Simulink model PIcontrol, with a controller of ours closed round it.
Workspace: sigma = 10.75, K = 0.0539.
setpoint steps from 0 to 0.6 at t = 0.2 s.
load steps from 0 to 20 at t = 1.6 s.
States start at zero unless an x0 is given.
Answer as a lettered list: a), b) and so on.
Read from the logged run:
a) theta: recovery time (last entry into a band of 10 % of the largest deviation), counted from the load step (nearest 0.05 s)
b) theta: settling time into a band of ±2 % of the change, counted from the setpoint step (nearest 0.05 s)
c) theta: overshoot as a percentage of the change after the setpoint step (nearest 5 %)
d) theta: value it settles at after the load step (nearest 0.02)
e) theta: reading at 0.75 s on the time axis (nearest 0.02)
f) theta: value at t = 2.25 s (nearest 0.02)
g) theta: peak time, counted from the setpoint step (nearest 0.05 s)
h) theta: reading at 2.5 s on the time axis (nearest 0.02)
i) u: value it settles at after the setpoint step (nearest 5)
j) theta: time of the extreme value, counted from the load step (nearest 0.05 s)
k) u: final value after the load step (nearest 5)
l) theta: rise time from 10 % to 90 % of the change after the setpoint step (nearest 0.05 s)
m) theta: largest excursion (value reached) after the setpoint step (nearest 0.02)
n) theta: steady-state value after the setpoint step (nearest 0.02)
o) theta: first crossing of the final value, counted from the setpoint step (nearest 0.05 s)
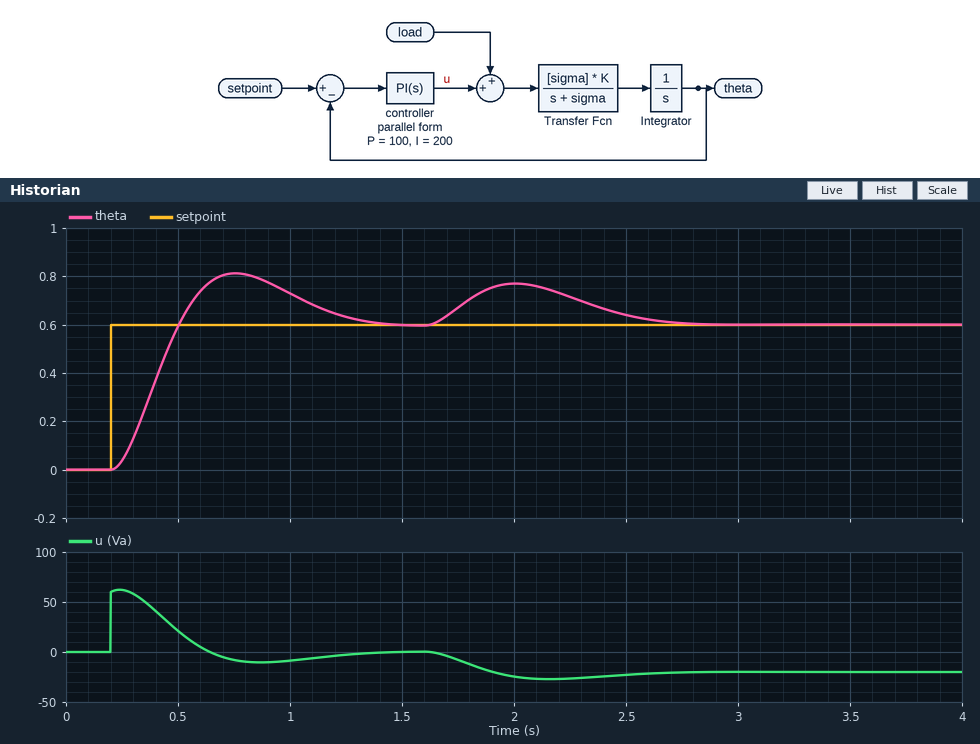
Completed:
a) 1.05 s
b) 1.15 s
c) 35 %
d) 0.60
e) 0.82
f) 0.72
g) 0.55 s
h) 0.64
i) 0
j) 0.40 s
k) -20
l) 0.20 s
m) 0.82
n) 0.60
o) 0.30 s
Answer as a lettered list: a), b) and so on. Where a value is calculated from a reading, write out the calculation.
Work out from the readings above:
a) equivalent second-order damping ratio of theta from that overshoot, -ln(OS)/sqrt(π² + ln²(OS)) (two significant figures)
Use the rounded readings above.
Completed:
a) ln(0.35) = -1.050; 1.050 / sqrt(9.870 + 1.102) = 0.32
